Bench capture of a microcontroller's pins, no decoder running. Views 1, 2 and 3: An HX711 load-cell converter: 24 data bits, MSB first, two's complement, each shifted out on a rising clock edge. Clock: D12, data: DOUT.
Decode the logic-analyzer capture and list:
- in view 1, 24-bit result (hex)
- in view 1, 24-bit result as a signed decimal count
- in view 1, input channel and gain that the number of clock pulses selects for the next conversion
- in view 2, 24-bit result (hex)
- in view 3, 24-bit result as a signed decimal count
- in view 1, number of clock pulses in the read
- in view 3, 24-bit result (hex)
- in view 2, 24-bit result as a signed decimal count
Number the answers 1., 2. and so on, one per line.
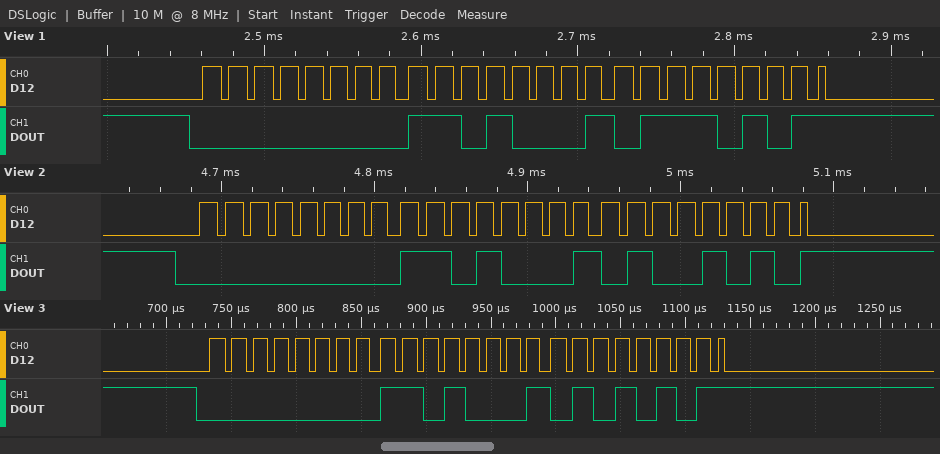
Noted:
1. 0x00D175
2. 53621
3. channel A, gain 128
4. 0x00D14A
5. 53589
6. 25
7. 0x00D155
8. 53578
